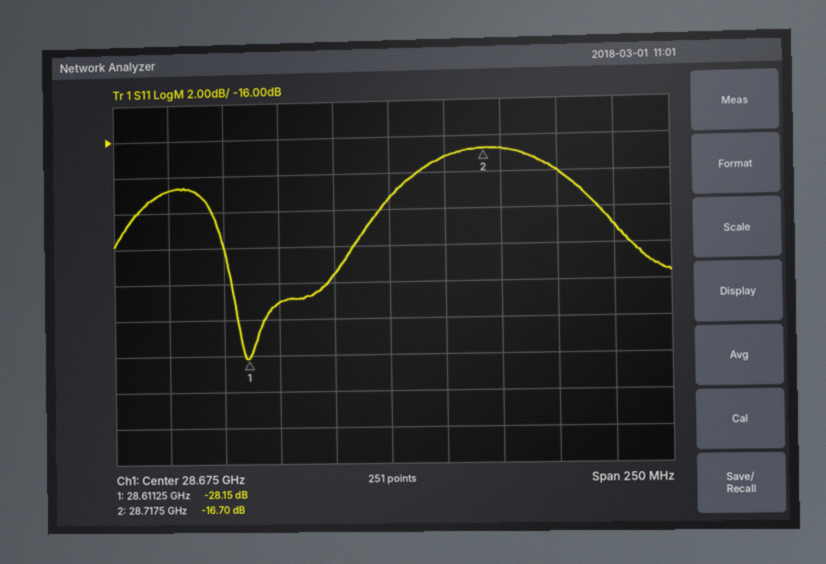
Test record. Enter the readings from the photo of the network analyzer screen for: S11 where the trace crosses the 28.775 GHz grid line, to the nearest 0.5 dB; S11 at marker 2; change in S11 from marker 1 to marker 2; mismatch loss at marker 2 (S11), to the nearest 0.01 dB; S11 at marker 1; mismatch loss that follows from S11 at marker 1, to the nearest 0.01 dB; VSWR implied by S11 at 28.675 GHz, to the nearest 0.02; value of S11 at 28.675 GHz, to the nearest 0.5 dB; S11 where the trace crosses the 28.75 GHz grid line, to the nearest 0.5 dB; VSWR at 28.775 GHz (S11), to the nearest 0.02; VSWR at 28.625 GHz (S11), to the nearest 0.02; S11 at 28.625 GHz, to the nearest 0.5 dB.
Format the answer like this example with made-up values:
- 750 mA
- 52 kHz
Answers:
- -21.0 dB
- -16.70 dB
- 11.45 dB
- 0.09 dB
- -28.15 dB
- 0.01 dB
- 1.24
- -19.5 dB
- -18.0 dB
- 1.20
- 1.12
- -25.0 dB
